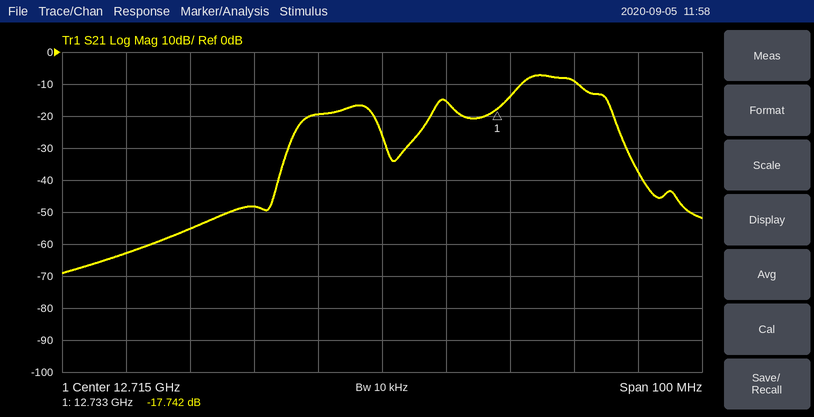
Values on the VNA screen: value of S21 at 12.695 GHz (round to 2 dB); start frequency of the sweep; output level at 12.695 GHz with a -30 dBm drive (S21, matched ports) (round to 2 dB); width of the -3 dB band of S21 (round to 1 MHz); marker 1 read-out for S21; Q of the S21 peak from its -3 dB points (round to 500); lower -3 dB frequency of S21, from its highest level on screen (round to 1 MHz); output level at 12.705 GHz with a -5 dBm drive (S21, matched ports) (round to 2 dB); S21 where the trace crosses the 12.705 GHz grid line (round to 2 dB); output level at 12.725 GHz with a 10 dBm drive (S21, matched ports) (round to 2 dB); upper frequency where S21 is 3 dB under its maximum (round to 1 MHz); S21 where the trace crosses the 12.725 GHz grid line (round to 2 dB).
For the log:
-48 dB
12.665 GHz
-78 dBm
9 MHz
-17.742 dB
1500
12.737 GHz
-24 dBm
-20 dB
-6 dBm
12.746 GHz
-16 dB
